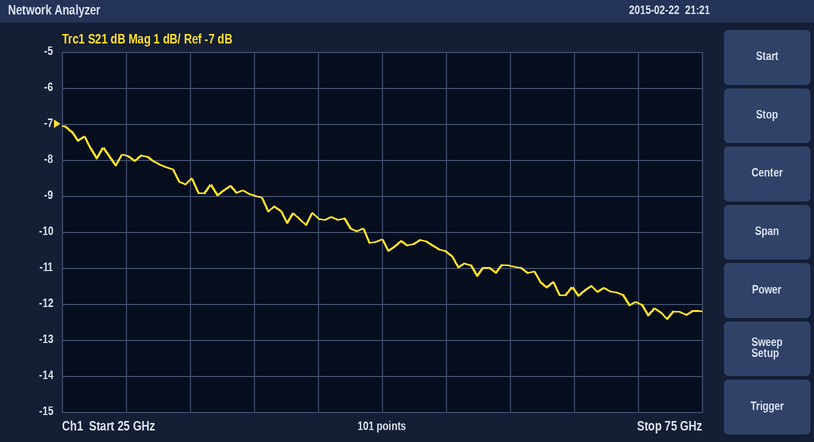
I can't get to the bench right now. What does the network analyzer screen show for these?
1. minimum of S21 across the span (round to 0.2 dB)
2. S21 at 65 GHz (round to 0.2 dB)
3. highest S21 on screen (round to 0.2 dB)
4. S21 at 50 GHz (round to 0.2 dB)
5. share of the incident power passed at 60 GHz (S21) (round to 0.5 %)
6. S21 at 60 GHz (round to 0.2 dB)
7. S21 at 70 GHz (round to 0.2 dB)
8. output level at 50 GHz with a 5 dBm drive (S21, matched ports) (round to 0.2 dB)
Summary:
-12.4 dB
-11.6 dB
-7.0 dB
-10.2 dB
8.0 %
-11.0 dB
-12.0 dB
-5.2 dBm
